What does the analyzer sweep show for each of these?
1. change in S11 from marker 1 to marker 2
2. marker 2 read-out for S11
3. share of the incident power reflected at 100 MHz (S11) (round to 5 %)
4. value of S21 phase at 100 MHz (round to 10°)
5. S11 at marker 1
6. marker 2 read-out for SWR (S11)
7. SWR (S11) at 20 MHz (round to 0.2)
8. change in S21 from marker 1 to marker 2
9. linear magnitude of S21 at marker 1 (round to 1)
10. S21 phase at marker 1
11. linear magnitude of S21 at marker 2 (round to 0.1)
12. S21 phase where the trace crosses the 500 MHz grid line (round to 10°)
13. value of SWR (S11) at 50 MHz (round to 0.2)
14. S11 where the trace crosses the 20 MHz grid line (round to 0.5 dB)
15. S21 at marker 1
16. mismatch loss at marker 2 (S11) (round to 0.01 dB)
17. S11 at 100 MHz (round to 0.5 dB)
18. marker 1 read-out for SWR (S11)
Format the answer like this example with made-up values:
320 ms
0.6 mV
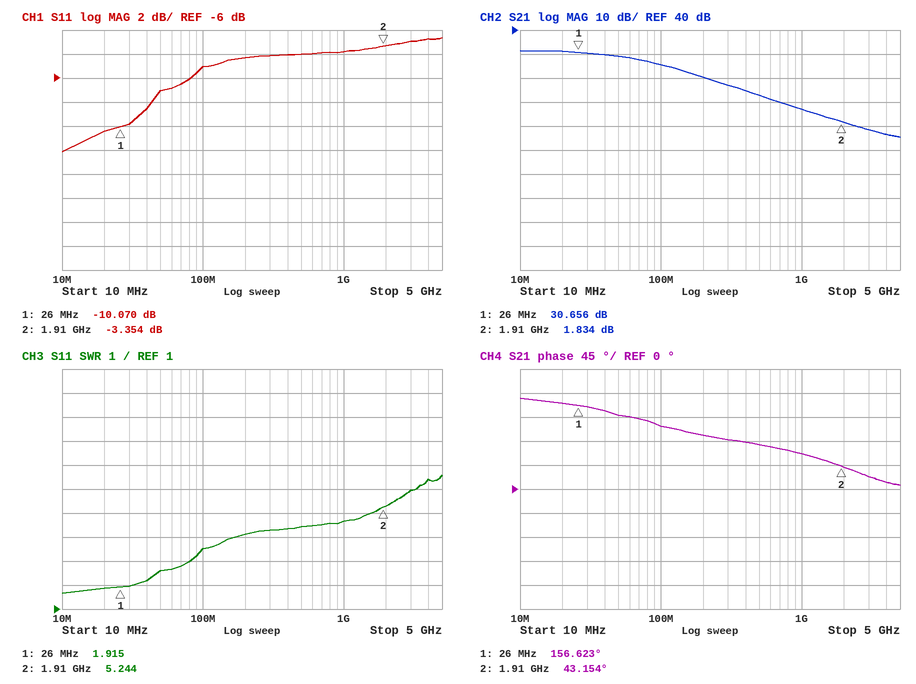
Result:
6.716 dB
-3.354 dB
30 %
120°
-10.070 dB
5.244
1.8
-28.822 dB
34
156.623°
1.2
80°
2.6
-10.5 dB
30.656 dB
2.69 dB
-5.0 dB
1.915
